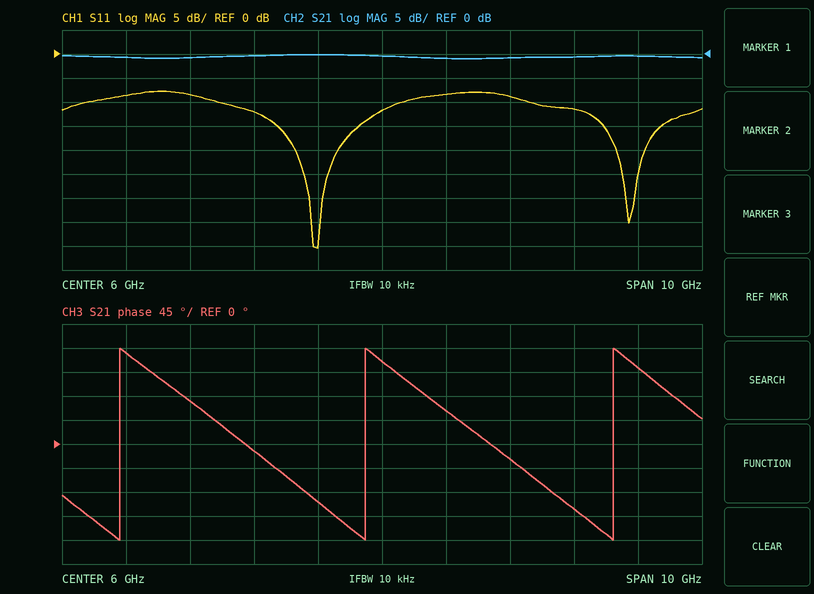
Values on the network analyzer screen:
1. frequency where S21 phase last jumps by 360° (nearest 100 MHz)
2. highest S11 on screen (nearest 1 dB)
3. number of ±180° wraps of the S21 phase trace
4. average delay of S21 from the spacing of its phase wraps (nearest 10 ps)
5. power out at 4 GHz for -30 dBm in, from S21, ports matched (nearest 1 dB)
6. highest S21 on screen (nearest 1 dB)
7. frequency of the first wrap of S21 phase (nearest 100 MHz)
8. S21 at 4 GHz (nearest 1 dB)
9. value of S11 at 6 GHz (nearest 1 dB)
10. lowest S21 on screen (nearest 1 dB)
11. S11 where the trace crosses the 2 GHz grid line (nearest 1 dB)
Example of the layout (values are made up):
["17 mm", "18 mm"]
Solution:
["9.6 GHz", "-8 dB", "3", "260 ps", "-30 dBm", "0 dB", "1.9 GHz", "0 dB", "-12 dB", "-1 dB", "-9 dB"]
